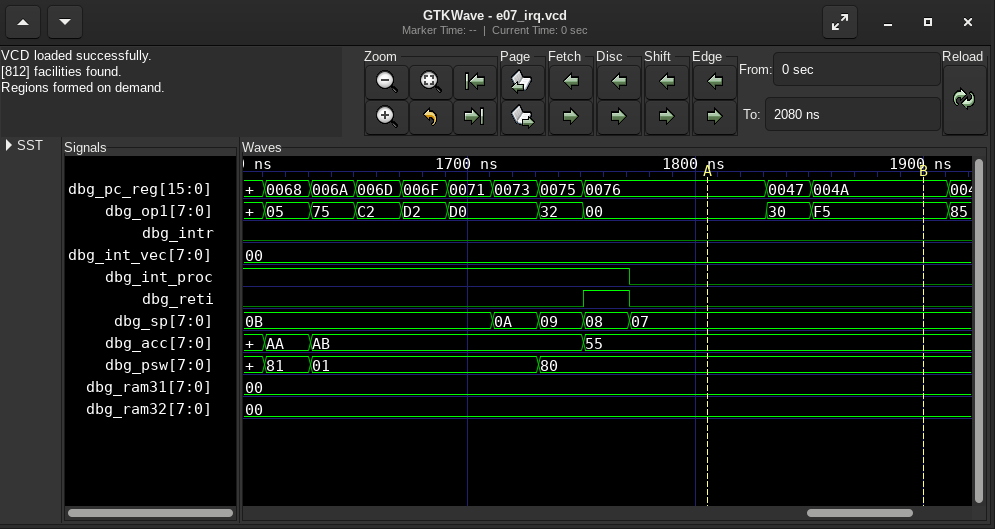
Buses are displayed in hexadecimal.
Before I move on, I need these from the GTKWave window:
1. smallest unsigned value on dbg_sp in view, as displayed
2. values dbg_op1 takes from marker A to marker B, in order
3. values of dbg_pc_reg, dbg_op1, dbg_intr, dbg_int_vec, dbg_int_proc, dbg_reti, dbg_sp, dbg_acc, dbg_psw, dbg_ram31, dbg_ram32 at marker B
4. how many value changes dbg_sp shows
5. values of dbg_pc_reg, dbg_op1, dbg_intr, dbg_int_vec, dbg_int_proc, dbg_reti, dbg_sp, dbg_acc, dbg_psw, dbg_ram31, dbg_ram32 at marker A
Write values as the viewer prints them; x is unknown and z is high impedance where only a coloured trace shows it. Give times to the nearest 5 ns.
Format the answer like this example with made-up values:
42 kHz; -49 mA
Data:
07; 00, 30, F5; dbg_pc_reg=004A, dbg_op1=F5, dbg_intr=0, dbg_int_vec=00, dbg_int_proc=0, dbg_reti=0, dbg_sp=07, dbg_acc=55, dbg_psw=80, dbg_ram31=00, dbg_ram32=00; 4; dbg_pc_reg=0076, dbg_op1=00, dbg_intr=0, dbg_int_vec=00, dbg_int_proc=0, dbg_reti=0, dbg_sp=07, dbg_acc=55, dbg_psw=80, dbg_ram31=00, dbg_ram32=00
